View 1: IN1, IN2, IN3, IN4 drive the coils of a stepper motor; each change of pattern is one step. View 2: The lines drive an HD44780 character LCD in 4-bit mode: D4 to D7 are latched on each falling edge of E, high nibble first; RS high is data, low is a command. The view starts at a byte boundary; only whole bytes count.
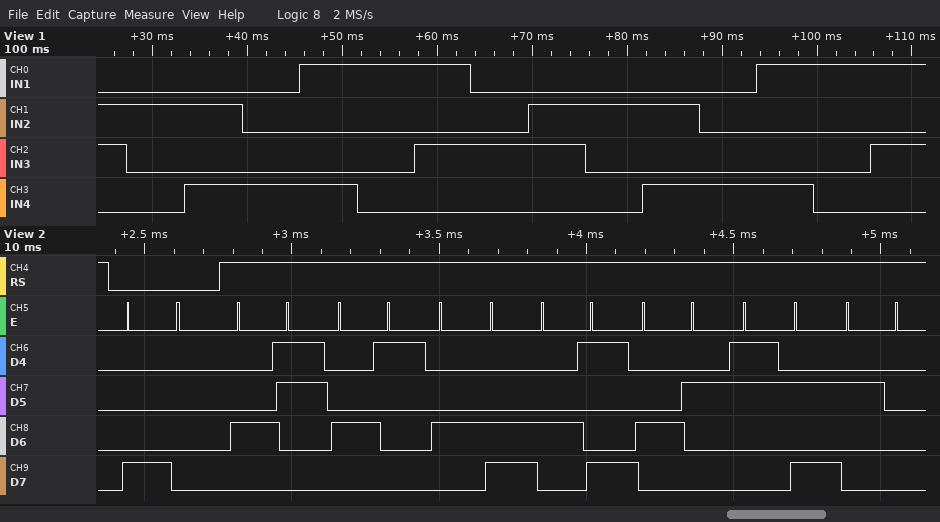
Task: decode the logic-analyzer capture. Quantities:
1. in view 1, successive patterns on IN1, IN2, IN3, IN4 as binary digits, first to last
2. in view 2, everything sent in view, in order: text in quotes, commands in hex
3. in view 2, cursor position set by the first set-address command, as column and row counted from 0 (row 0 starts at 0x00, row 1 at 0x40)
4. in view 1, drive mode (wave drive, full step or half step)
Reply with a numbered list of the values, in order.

1. 0110 0100 0101 0001 1001 1000 1010 0010 0110 0100 0101 0001 1001 1000 1010
2. 0x80 "CALIB: "
3. column 0, row 0
4. half step
